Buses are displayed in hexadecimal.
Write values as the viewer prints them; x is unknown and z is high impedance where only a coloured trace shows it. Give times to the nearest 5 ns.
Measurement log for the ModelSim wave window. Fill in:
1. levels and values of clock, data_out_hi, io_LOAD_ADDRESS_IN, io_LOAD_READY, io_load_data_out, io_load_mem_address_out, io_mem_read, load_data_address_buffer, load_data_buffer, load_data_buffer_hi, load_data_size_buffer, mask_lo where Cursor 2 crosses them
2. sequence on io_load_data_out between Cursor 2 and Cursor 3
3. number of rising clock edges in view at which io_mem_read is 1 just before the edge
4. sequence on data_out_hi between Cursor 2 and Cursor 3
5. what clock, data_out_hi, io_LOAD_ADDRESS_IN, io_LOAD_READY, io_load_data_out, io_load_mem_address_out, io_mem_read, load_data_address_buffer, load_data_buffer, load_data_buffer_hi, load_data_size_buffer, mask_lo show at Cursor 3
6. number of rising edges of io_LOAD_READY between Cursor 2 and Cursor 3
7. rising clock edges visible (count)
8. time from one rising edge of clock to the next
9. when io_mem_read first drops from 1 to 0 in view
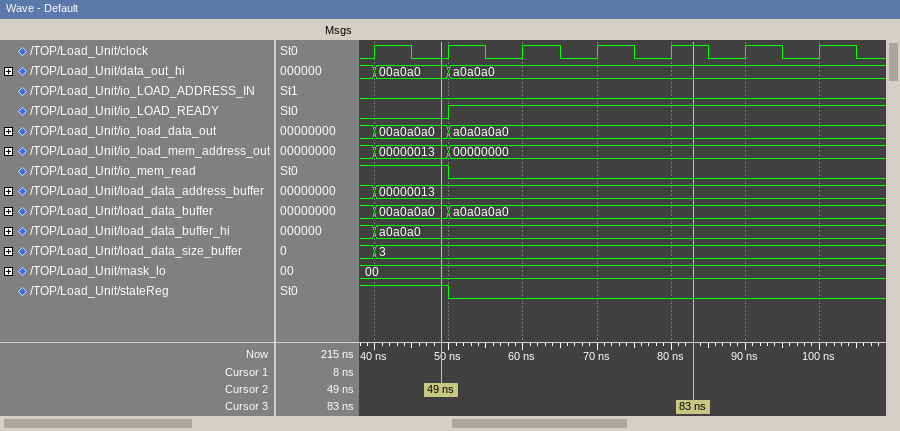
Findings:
clock=0, data_out_hi=00a0a0, io_LOAD_ADDRESS_IN=0, io_LOAD_READY=0, io_load_data_out=00a0a0a0, io_load_mem_address_out=00000013, io_mem_read=1, load_data_address_buffer=00000013, load_data_buffer=00a0a0a0, load_data_buffer_hi=a0a0a0, load_data_size_buffer=3, mask_lo=00
00a0a0a0, a0a0a0a0
2
00a0a0, a0a0a0
clock=1, data_out_hi=a0a0a0, io_LOAD_ADDRESS_IN=0, io_LOAD_READY=1, io_load_data_out=a0a0a0a0, io_load_mem_address_out=00000000, io_mem_read=0, load_data_address_buffer=00000013, load_data_buffer=a0a0a0a0, load_data_buffer_hi=a0a0a0, load_data_size_buffer=3, mask_lo=00
1
7
10 ns
50 ns
